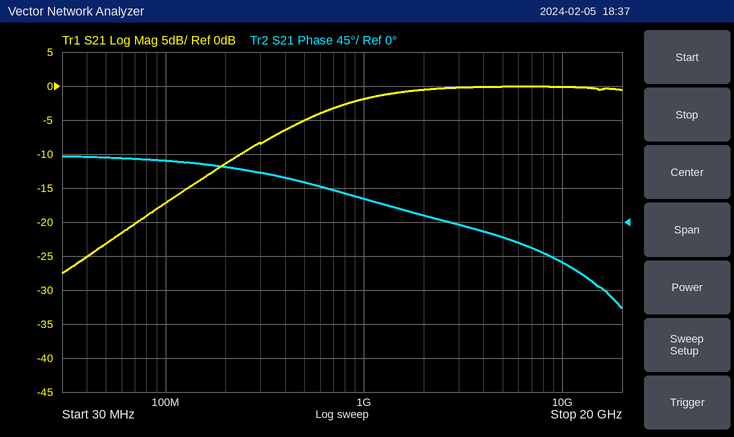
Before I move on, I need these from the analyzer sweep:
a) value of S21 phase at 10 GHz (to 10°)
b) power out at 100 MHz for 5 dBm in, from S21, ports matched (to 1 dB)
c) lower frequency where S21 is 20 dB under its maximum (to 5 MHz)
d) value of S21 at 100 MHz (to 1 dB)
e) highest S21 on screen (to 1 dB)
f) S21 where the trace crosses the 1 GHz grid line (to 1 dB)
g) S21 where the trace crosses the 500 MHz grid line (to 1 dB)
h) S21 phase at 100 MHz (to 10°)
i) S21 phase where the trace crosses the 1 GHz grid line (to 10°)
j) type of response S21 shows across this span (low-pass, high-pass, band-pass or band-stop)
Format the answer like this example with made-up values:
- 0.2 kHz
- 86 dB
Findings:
- -50°
- -12 dBm
- 70 MHz
- -17 dB
- 0 dB
- -2 dB
- -5 dB
- 80°
- 30°
- high-pass
